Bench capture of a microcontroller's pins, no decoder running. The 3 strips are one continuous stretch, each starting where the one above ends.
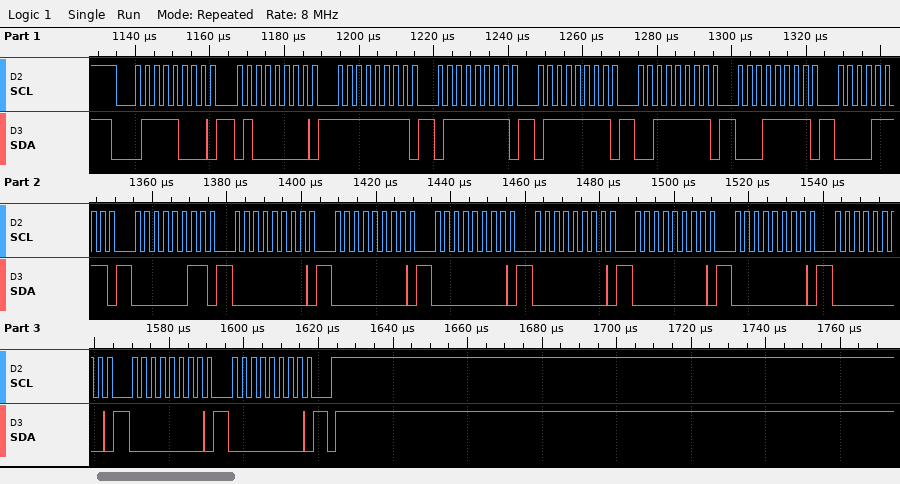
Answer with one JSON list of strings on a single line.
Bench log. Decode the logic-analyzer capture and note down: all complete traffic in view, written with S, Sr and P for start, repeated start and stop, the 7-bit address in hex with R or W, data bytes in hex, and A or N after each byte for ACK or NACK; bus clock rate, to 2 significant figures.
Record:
["S 3CW A 40 A FF A 7F A 7F A 3F A 1F A 0F A 03 A 00 A 00 A 00 A 00 A 00 A 00 A 00 A 00 A 00 A P", "400 kHz"]
